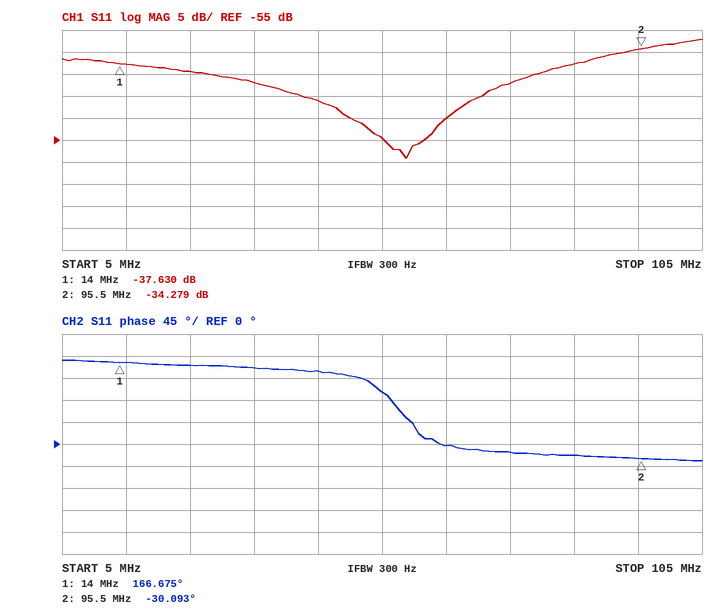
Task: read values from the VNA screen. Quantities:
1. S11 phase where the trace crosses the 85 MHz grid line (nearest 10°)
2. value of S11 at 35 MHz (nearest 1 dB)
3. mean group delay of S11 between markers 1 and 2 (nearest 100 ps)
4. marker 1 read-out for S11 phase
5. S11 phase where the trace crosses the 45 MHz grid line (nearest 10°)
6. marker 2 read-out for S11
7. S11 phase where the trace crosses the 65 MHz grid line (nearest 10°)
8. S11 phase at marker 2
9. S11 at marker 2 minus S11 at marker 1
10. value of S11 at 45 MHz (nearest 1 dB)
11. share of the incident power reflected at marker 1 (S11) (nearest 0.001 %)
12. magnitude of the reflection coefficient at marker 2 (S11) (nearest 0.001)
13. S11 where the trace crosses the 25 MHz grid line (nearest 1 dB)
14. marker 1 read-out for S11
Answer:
-20°
-42 dB
6.7 ns
166.675°
150°
-34.279 dB
0°
-30.093°
3.351 dB
-46 dB
0.017 %
0.019
-39 dB
-37.630 dB
